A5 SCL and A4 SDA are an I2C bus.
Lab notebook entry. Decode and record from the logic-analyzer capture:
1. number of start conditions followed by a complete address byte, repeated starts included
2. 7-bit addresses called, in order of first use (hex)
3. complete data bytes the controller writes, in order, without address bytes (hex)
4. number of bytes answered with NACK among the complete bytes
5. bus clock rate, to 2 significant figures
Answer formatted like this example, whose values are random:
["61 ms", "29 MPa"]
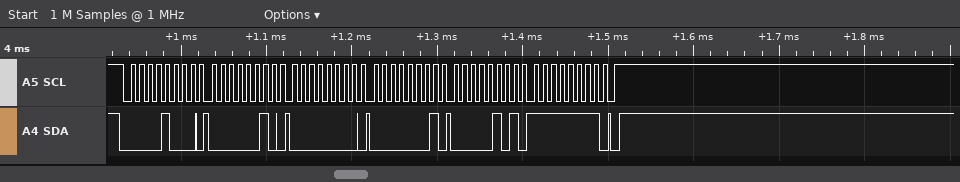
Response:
["1", "0x04", "02 00 01 05 FF", "0", "100 kHz"]
